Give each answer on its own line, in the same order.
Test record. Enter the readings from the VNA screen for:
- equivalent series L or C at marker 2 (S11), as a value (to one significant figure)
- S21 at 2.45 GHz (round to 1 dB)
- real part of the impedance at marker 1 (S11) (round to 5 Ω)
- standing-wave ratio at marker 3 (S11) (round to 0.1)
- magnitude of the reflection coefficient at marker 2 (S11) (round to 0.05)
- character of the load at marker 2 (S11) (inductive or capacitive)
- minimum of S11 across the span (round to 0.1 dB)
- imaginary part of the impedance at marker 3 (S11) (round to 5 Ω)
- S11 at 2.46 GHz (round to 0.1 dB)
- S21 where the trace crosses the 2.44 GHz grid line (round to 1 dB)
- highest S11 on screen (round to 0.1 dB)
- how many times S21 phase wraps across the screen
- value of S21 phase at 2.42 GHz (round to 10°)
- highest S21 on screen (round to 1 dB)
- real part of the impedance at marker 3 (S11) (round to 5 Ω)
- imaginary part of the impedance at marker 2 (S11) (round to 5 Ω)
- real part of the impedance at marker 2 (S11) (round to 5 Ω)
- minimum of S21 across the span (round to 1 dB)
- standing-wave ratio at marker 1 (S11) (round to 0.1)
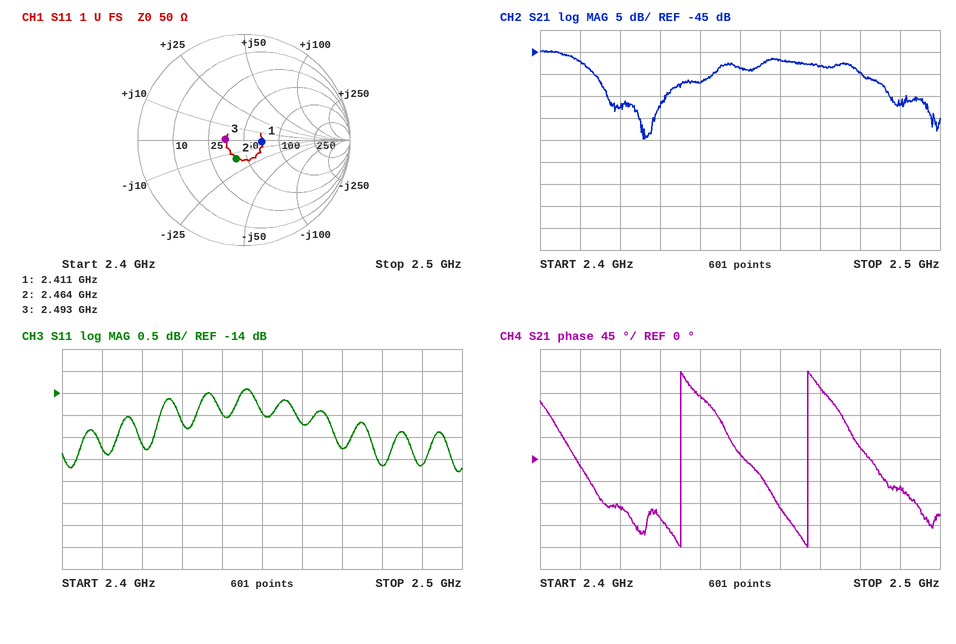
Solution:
4 pF
-49 dB
70 Ω
1.4
0.20
capacitive
-15.8 dB
0 Ω
-14.7 dB
-52 dB
-13.9 dB
2
-100°
-45 dB
35 Ω
-15 Ω
40 Ω
-65 dB
1.4
